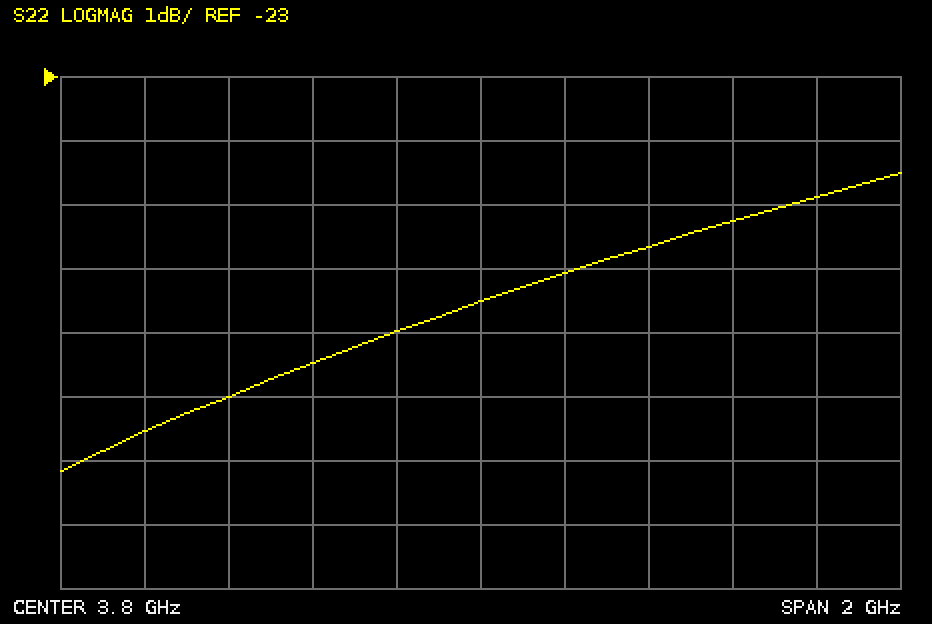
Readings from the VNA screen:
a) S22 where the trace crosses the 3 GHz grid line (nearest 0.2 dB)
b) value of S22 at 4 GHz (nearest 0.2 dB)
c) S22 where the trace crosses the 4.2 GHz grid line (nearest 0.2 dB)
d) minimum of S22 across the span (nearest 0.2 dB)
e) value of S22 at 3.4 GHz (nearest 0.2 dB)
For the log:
-28.6 dB
-26.0 dB
-25.6 dB
-29.2 dB
-27.4 dB
